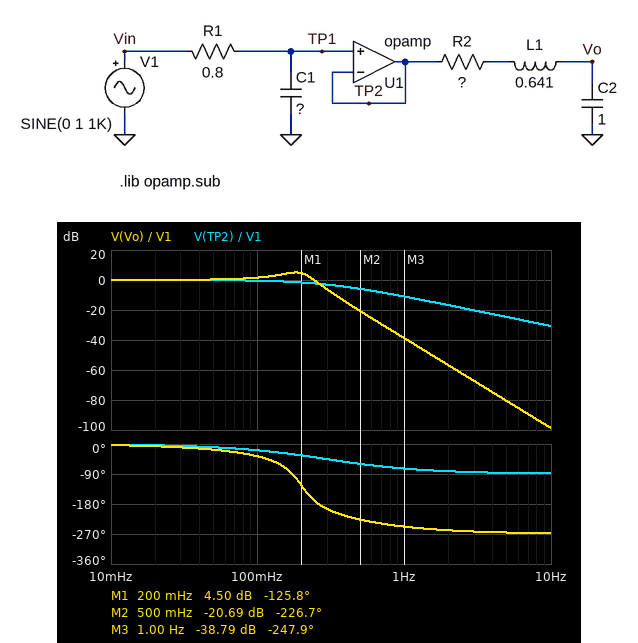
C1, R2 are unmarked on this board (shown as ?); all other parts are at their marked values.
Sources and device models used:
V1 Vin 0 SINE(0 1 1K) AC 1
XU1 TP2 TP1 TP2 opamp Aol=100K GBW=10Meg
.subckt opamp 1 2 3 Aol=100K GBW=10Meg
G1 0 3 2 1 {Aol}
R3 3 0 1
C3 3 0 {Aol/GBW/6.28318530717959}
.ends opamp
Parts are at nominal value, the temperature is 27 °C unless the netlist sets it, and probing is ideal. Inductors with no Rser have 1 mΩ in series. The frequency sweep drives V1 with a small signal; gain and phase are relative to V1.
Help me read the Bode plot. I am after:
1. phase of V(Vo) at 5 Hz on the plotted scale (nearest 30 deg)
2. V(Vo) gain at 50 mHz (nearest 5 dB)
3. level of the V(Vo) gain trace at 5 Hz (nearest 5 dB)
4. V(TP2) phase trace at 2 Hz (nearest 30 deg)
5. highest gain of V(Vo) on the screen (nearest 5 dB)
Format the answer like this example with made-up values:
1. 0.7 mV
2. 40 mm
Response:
1. -270 deg
2. 0 dB
3. -80 dB
4. -90 deg
5. 5 dB
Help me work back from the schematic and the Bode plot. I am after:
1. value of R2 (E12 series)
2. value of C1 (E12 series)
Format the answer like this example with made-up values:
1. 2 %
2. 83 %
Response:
1. 0.39 Ω
2. 680 mF
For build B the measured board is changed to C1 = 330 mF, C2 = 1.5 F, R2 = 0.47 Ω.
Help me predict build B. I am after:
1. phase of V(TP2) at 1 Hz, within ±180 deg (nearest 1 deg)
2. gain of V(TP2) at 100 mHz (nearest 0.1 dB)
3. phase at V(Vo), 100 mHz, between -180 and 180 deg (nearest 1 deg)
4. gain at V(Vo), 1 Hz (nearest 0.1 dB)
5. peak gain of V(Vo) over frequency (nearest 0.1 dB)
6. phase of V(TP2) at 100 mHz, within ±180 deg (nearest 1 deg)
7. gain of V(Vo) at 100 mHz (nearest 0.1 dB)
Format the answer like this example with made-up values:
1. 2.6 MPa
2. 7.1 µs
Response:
1. -59 deg
2. -0.1 dB
3. -45 deg
4. -37.2 dB
5. 3.2 dB
6. -9 deg
7. 2.2 dB
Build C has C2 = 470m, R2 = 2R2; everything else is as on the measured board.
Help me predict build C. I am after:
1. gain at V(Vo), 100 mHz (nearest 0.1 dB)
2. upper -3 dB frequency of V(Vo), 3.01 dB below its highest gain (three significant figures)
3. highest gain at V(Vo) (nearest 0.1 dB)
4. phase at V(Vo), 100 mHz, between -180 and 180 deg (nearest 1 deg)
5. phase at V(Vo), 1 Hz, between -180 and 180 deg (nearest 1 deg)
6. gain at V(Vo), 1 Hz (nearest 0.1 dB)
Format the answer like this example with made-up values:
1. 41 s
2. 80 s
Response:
1. -1.3 dB
2. 158 mHz
3. 0 dB
4. -55 deg
5. 137 deg
6. -33.1 dB
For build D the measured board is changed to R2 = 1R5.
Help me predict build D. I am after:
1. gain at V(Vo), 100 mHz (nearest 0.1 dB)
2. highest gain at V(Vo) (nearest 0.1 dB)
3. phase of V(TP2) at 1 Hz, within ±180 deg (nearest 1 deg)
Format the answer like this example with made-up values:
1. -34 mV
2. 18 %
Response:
1. -2.1 dB
2. 0 dB
3. -74 deg
